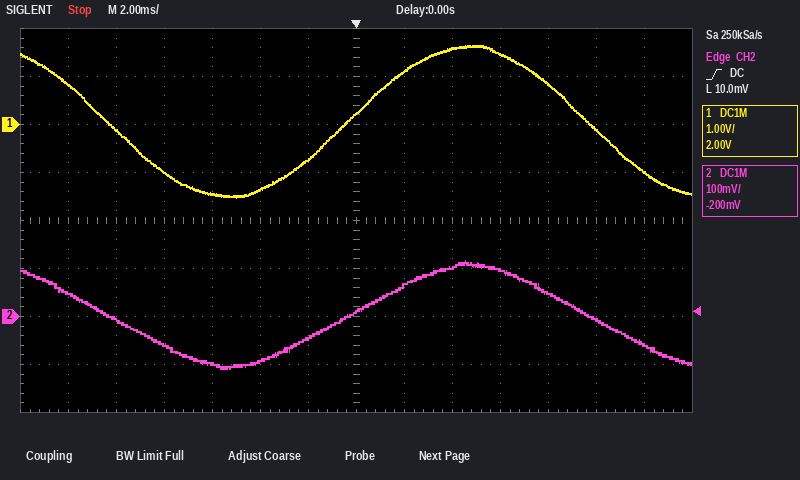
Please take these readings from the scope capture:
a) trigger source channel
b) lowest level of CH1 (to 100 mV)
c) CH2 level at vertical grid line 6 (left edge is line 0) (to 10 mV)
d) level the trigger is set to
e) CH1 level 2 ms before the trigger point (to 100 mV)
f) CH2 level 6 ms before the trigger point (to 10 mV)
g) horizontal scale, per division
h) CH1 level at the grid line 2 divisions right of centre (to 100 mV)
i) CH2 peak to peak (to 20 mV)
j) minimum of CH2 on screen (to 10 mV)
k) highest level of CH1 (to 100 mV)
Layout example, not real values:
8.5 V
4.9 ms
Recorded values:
CH2
-1.5 V
-40 mV
10.0 mV
-700 mV
-100 mV
2 ms
1.6 V
220 mV
-110 mV
1.6 V
